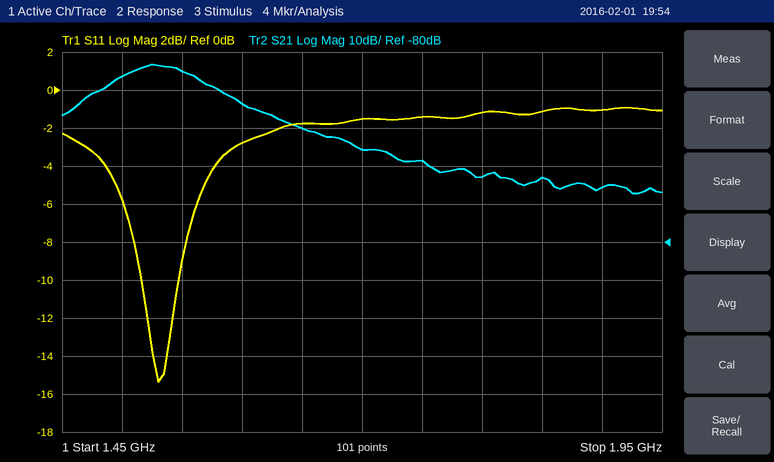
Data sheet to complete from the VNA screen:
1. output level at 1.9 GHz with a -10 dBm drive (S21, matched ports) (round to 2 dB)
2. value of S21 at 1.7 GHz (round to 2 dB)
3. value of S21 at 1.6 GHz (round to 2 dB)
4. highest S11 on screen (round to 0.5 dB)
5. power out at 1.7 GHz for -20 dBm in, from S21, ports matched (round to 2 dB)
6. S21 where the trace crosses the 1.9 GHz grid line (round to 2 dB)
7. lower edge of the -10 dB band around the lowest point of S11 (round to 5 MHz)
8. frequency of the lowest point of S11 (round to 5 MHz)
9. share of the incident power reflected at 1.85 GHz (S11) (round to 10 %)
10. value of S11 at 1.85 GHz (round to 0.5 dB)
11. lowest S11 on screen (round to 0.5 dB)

-76 dBm
-56 dB
-44 dB
-1.0 dB
-76 dBm
-66 dB
1.515 GHz
1.530 GHz
80 %
-1.0 dB
-15.5 dB
